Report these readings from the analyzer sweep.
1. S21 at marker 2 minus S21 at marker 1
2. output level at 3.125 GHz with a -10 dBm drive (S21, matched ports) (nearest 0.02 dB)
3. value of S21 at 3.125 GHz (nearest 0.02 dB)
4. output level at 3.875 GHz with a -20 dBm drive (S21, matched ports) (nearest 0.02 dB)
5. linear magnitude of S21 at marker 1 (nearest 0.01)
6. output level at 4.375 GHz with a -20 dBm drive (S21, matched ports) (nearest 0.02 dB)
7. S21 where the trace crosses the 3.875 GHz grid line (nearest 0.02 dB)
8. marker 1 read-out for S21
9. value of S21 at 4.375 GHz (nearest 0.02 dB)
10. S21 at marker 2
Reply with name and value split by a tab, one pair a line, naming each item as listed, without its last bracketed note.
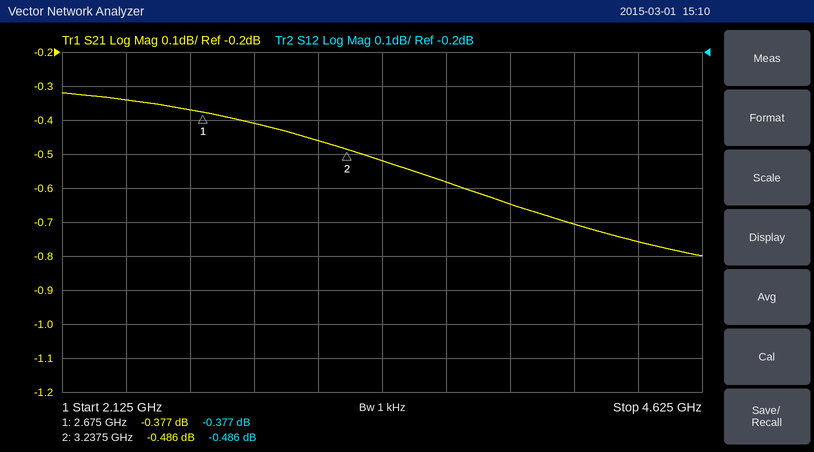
S21 at marker 2 minus S21 at marker 1	-0.109 dB
output level at 3.125 GHz with a -10 dBm drive (S21, matched ports)	-10.46 dBm
value of S21 at 3.125 GHz	-0.46 dB
output level at 3.875 GHz with a -20 dBm drive (S21, matched ports)	-20.64 dBm
linear magnitude of S21 at marker 1	0.96
output level at 4.375 GHz with a -20 dBm drive (S21, matched ports)	-20.76 dBm
S21 where the trace crosses the 3.875 GHz grid line	-0.64 dB
marker 1 read-out for S21	-0.377 dB
value of S21 at 4.375 GHz	-0.76 dB
S21 at marker 2	-0.486 dB
